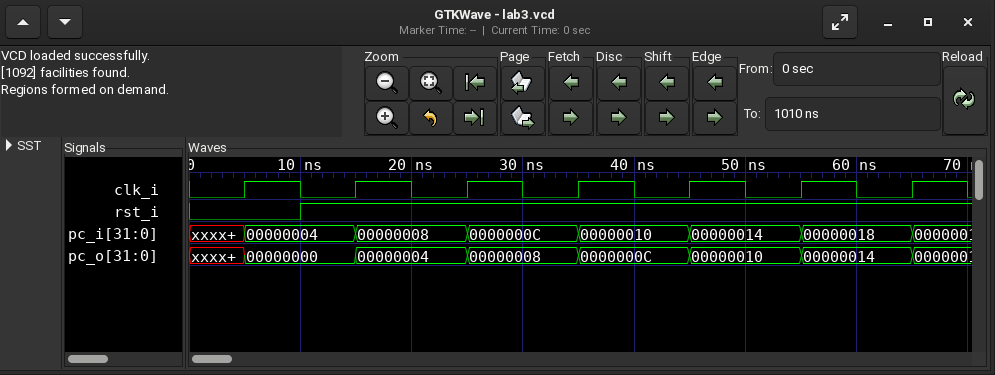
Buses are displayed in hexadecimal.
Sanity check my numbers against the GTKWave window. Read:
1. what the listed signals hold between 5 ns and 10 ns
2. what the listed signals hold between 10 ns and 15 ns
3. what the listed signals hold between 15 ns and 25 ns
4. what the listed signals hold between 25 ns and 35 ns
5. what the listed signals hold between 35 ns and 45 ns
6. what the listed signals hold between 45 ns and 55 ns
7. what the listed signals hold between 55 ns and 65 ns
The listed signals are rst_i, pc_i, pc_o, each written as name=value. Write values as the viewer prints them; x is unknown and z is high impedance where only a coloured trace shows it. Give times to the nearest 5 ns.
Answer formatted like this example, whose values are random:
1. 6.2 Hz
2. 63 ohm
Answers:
1. rst_i=0, pc_i=00000004, pc_o=00000000
2. rst_i=1, pc_i=00000004, pc_o=00000000
3. rst_i=1, pc_i=00000008, pc_o=00000004
4. rst_i=1, pc_i=0000000C, pc_o=00000008
5. rst_i=1, pc_i=00000010, pc_o=0000000C
6. rst_i=1, pc_i=00000014, pc_o=00000010
7. rst_i=1, pc_i=00000018, pc_o=00000014
